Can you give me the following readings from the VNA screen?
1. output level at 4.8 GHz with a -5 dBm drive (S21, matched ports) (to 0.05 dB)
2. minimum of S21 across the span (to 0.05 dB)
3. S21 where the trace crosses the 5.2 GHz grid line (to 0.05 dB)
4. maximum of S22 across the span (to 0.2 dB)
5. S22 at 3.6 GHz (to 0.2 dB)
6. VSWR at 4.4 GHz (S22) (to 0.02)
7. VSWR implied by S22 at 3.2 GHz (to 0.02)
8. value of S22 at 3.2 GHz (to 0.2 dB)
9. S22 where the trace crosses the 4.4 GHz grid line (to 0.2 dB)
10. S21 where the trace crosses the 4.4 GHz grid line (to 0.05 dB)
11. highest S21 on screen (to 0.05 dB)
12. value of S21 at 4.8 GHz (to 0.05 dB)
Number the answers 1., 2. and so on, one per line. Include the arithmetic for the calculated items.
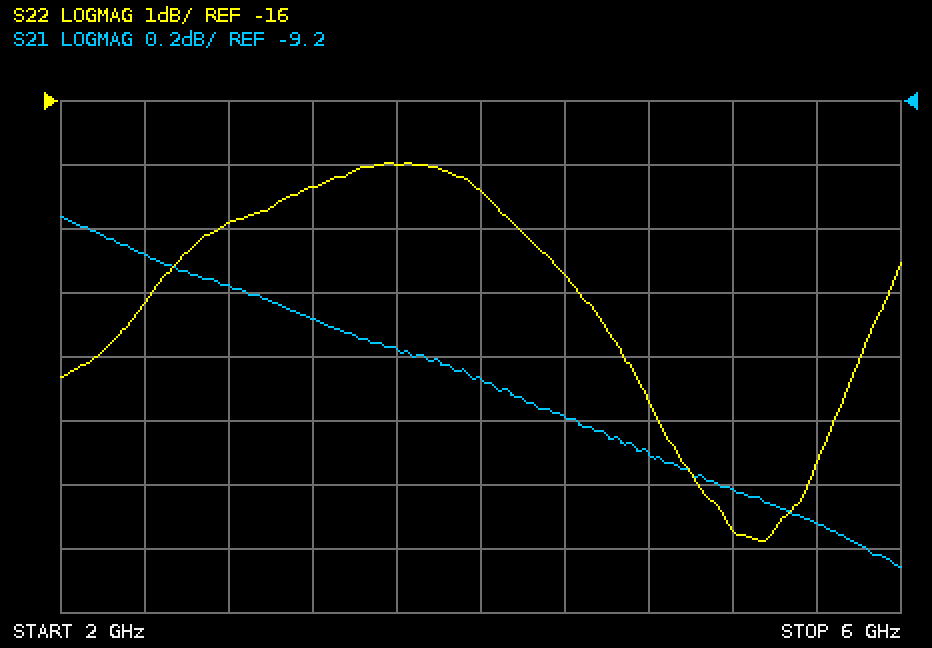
1. -5 dBm + (-10.30 dB) = -15.30 dBm
2. -10.65 dB
3. -10.40 dB
4. -17.0 dB
5. -17.0 dB
6. |Γ| = 10^(-18.8/20) = 0.1148; VSWR = (1 + 0.1148)/(1 − 0.1148) ≈ 1.26
7. |Γ| = 10^(-17.4/20) = 0.1349; VSWR = (1 + 0.1349)/(1 − 0.1349) ≈ 1.31, so 1.32 to the nearest 0.02
8. -17.4 dB
9. -18.8 dB
10. -10.20 dB
11. -9.55 dB
12. -10.30 dB
